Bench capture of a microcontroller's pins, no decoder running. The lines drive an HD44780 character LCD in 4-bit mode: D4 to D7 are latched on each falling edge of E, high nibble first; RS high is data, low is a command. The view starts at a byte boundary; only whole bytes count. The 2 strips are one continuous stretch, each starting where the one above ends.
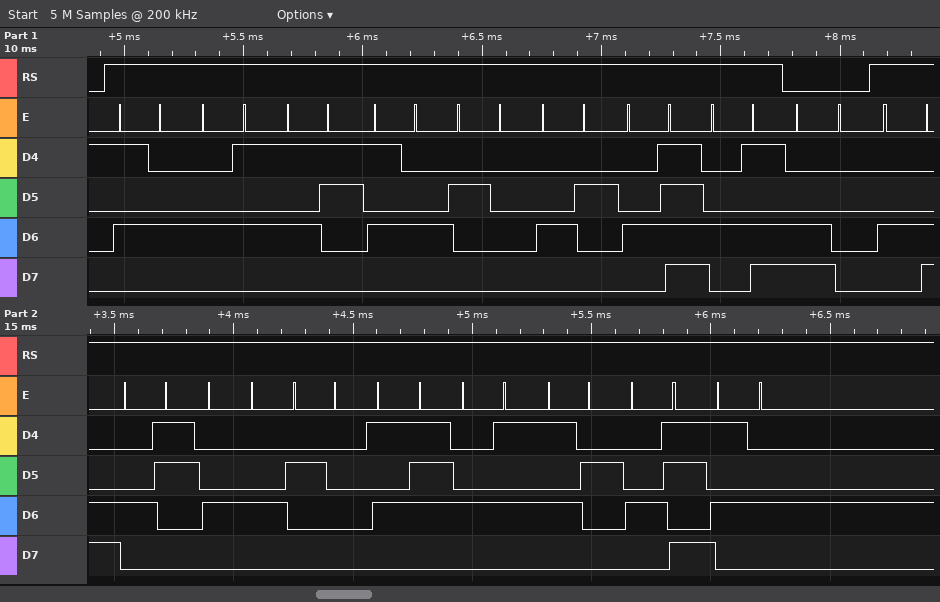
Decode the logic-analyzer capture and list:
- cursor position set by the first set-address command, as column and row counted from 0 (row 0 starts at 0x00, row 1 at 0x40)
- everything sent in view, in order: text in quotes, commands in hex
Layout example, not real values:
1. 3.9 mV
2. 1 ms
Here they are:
1. column 0, row 1
2. "TEST BOM" 0xC0 "LCD WERKT"
